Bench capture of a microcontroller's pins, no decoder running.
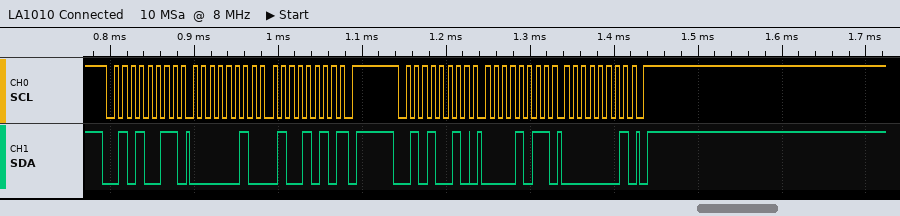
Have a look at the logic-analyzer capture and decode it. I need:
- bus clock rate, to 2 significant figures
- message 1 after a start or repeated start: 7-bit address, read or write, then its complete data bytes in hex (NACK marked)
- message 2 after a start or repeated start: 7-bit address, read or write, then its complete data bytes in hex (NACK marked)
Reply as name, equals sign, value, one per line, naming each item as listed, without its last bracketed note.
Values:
bus clock rate, to 2 significant figures = 100 kHz
message 1 after a start or repeated start: 7-bit address, read or write, then its complete data bytes in hex = 0x29 read: 02 4A NACK
message 2 after a start or repeated start: 7-bit address, read or write, then its complete data bytes in hex = 0x29 write: 0B 01
